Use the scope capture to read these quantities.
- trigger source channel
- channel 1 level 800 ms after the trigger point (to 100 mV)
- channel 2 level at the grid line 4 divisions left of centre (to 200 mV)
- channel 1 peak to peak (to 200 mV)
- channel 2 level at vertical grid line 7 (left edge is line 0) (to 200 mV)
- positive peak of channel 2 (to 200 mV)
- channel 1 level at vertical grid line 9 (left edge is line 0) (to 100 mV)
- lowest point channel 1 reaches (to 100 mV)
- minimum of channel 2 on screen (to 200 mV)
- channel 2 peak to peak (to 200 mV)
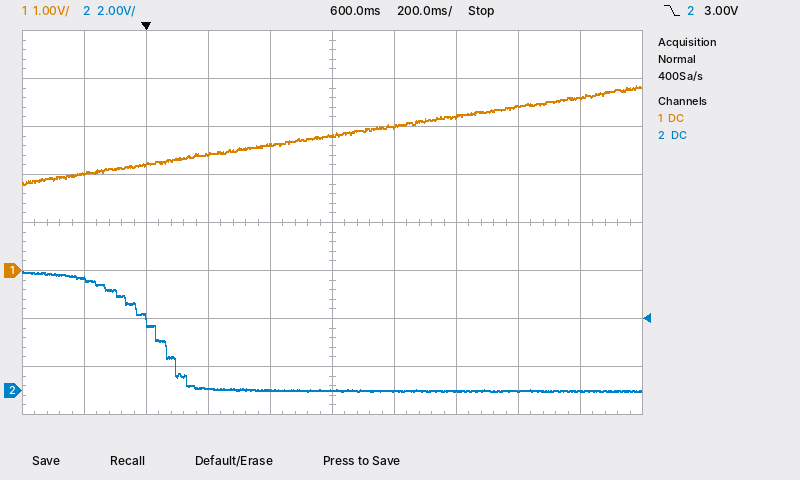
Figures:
channel 2
3.0 V
4.6 V
2.0 V
0.0 V
5.0 V
3.6 V
1.8 V
0.0 V
5.0 V
